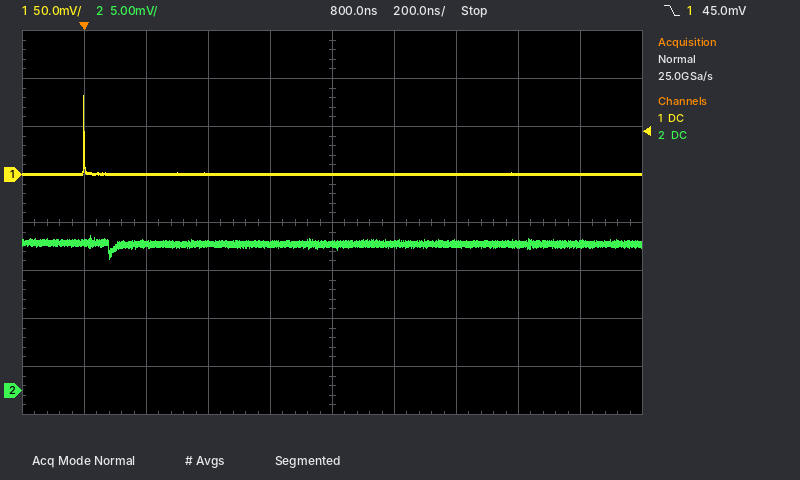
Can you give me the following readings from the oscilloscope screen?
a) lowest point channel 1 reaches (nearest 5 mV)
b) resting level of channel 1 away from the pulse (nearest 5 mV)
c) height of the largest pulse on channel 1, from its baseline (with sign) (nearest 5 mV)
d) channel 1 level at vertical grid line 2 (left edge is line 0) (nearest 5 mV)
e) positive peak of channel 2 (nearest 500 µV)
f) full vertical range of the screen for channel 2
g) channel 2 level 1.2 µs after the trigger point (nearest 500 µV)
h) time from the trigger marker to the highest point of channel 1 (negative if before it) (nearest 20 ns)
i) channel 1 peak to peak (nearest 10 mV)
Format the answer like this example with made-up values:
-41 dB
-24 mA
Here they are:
0 mV
0 mV
+80 mV
0 mV
16.0 mV
40 mV
15.5 mV
0 ns
80 mV
